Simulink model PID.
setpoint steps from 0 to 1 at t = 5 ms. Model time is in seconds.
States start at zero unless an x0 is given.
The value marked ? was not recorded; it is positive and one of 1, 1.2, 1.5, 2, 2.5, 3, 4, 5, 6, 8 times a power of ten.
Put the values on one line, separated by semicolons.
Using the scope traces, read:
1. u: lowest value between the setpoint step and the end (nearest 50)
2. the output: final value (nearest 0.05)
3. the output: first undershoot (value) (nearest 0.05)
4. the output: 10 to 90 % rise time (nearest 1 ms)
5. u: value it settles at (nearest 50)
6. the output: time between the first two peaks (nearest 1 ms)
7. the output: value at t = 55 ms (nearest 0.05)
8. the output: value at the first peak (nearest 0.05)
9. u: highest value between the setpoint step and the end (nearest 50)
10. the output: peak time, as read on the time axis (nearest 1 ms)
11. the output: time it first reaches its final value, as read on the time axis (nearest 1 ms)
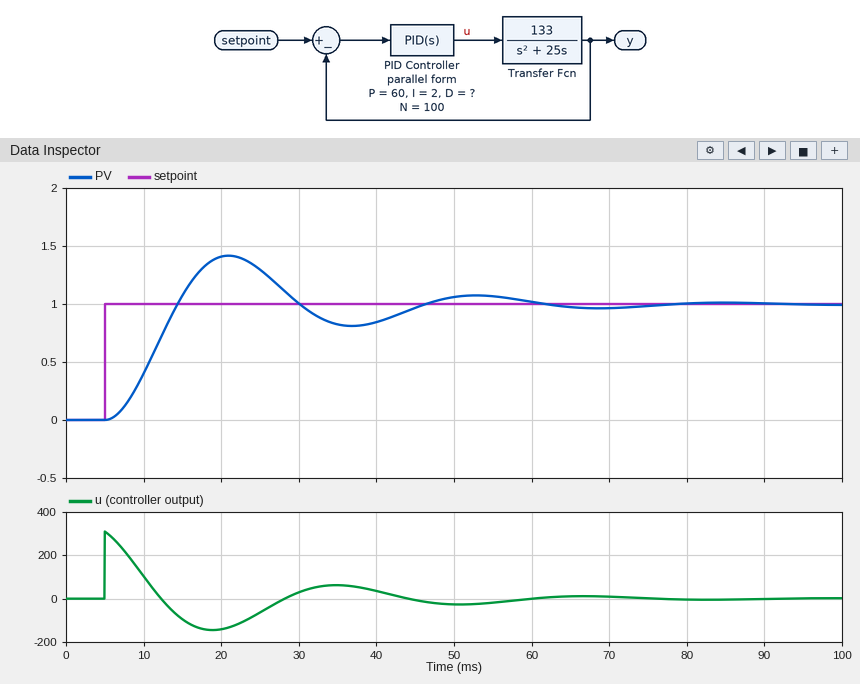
-150; 1.00; 0.80; 6 ms; 0; 32 ms; 1.05; 1.40; 300; 21 ms; 14 ms
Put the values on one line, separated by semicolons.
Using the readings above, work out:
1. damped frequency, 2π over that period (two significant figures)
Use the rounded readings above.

0.20 rad/ms
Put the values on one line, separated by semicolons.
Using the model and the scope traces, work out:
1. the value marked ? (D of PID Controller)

2.5
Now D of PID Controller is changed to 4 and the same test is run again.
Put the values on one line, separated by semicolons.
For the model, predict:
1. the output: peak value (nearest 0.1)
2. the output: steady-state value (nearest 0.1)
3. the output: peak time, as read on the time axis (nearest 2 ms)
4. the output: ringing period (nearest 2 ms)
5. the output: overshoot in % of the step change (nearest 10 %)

1.5; 1.0; 18 ms; 26 ms; 50 %
